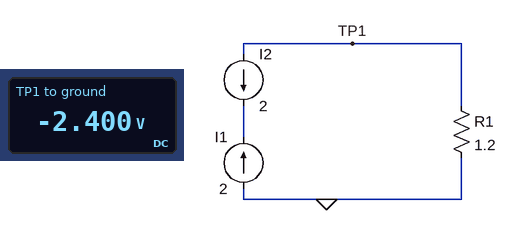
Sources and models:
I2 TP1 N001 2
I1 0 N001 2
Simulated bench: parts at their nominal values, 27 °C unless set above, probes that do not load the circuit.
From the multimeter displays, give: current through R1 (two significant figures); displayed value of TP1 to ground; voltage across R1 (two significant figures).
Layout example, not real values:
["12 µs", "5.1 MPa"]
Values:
["2.0 A", "-2.400 V", "2.4 V"]
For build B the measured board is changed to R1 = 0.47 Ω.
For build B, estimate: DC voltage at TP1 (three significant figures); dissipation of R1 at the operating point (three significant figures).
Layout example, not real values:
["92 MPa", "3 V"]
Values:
["-940 mV", "1.88 W"]
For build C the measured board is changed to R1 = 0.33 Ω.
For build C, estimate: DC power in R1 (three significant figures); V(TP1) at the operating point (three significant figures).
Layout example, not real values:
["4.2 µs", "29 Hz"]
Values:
["1.32 W", "-660 mV"]
